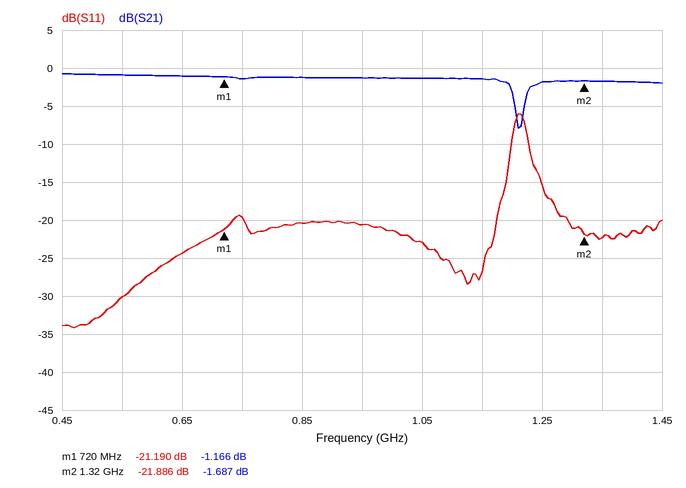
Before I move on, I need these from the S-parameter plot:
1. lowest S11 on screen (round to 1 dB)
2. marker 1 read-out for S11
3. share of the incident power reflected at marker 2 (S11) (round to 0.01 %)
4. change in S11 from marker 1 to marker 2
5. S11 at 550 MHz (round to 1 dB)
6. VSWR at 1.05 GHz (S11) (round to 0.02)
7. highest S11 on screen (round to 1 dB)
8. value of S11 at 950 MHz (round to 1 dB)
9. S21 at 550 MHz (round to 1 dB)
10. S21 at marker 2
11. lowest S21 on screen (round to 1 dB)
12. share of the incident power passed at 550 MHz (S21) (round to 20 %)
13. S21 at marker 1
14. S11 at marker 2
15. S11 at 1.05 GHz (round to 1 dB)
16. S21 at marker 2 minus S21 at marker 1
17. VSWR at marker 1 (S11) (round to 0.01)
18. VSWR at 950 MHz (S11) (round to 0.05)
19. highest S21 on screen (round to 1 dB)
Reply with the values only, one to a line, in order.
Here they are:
-34 dB
-21.190 dB
0.65 %
-0.696 dB
-30 dB
1.16
-6 dB
-21 dB
-1 dB
-1.687 dB
-8 dB
80 %
-1.166 dB
-21.886 dB
-23 dB
-0.521 dB
1.19
1.20
-1 dB
